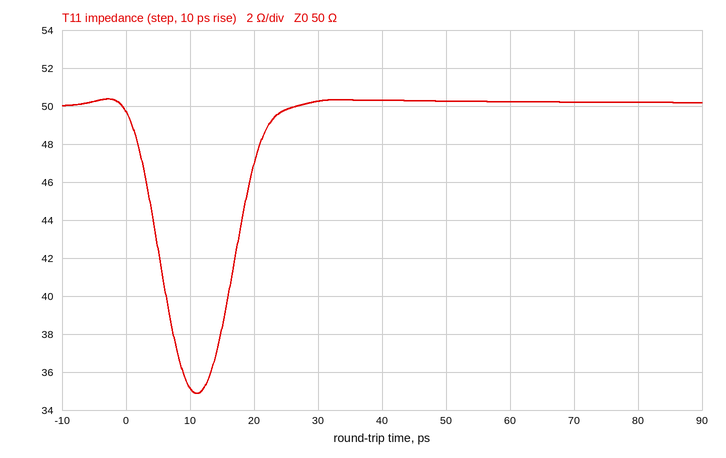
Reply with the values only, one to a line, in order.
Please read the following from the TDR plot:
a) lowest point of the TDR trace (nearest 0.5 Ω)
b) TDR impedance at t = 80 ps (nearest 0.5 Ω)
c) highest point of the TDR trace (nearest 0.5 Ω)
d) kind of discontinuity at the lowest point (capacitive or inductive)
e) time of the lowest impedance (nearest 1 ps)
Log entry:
35.0 Ω
50.0 Ω
50.5 Ω
capacitive
11 ps
